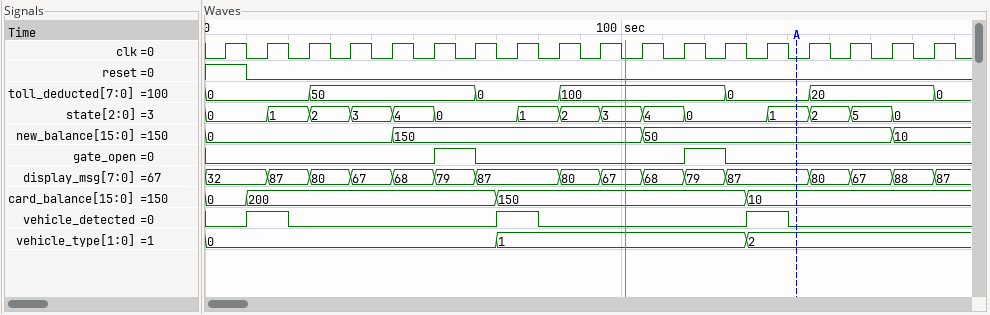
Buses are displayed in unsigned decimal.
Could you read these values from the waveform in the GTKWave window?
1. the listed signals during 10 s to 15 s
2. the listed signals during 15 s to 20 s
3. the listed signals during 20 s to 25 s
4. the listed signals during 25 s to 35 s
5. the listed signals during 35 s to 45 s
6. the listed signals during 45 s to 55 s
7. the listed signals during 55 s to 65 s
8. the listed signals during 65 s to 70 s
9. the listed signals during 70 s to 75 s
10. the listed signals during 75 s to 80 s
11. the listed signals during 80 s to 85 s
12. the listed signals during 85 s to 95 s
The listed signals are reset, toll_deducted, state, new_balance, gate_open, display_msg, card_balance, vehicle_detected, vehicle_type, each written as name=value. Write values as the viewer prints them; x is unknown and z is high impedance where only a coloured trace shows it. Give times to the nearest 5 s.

reset=0, toll_deducted=0, state=0, new_balance=0, gate_open=0, display_msg=32, card_balance=200, vehicle_detected=1, vehicle_type=0
reset=0, toll_deducted=0, state=1, new_balance=0, gate_open=0, display_msg=87, card_balance=200, vehicle_detected=1, vehicle_type=0
reset=0, toll_deducted=0, state=1, new_balance=0, gate_open=0, display_msg=87, card_balance=200, vehicle_detected=0, vehicle_type=0
reset=0, toll_deducted=50, state=2, new_balance=0, gate_open=0, display_msg=80, card_balance=200, vehicle_detected=0, vehicle_type=0
reset=0, toll_deducted=50, state=3, new_balance=0, gate_open=0, display_msg=67, card_balance=200, vehicle_detected=0, vehicle_type=0
reset=0, toll_deducted=50, state=4, new_balance=150, gate_open=0, display_msg=68, card_balance=200, vehicle_detected=0, vehicle_type=0
reset=0, toll_deducted=50, state=0, new_balance=150, gate_open=1, display_msg=79, card_balance=200, vehicle_detected=0, vehicle_type=0
reset=0, toll_deducted=0, state=0, new_balance=150, gate_open=0, display_msg=87, card_balance=200, vehicle_detected=0, vehicle_type=0
reset=0, toll_deducted=0, state=0, new_balance=150, gate_open=0, display_msg=87, card_balance=150, vehicle_detected=1, vehicle_type=1
reset=0, toll_deducted=0, state=1, new_balance=150, gate_open=0, display_msg=87, card_balance=150, vehicle_detected=1, vehicle_type=1
reset=0, toll_deducted=0, state=1, new_balance=150, gate_open=0, display_msg=87, card_balance=150, vehicle_detected=0, vehicle_type=1
reset=0, toll_deducted=100, state=2, new_balance=150, gate_open=0, display_msg=80, card_balance=150, vehicle_detected=0, vehicle_type=1
